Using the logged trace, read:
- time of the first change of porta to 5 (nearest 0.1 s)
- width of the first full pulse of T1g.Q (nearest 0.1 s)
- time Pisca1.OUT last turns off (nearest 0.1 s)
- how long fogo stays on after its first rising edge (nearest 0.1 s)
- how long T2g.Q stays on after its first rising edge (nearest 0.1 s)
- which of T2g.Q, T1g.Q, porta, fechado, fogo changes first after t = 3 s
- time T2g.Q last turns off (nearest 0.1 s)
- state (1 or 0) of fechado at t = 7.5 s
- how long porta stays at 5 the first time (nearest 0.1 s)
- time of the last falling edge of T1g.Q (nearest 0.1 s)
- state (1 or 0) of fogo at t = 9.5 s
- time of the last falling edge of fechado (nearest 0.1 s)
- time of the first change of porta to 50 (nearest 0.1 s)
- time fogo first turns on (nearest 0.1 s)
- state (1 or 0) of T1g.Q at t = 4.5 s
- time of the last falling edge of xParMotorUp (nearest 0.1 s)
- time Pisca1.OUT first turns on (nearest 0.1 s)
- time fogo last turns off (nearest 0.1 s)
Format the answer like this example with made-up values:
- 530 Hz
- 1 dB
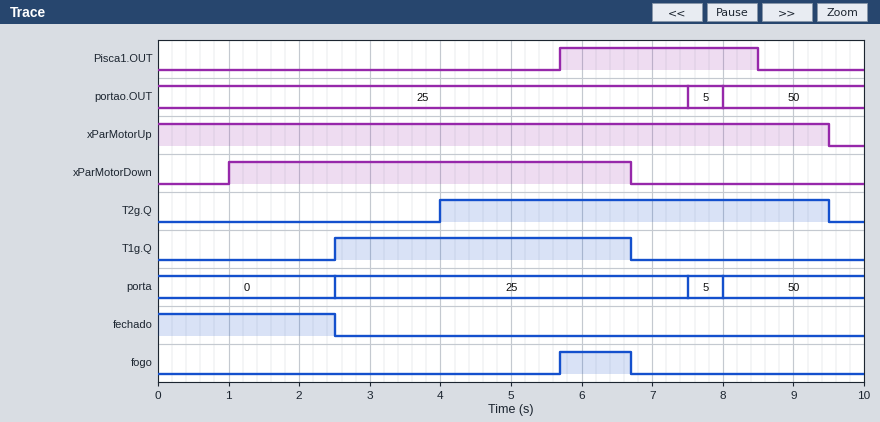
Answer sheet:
- 7.5 s
- 4.2 s
- 8.5 s
- 1.0 s
- 5.5 s
- T2g.Q
- 9.5 s
- 0
- 0.5 s
- 6.7 s
- 0
- 2.5 s
- 8.0 s
- 5.7 s
- 1
- 9.5 s
- 5.7 s
- 6.7 s
